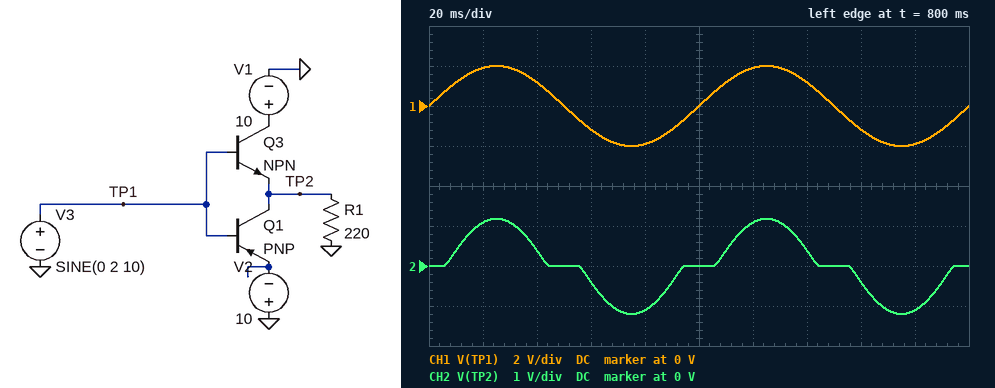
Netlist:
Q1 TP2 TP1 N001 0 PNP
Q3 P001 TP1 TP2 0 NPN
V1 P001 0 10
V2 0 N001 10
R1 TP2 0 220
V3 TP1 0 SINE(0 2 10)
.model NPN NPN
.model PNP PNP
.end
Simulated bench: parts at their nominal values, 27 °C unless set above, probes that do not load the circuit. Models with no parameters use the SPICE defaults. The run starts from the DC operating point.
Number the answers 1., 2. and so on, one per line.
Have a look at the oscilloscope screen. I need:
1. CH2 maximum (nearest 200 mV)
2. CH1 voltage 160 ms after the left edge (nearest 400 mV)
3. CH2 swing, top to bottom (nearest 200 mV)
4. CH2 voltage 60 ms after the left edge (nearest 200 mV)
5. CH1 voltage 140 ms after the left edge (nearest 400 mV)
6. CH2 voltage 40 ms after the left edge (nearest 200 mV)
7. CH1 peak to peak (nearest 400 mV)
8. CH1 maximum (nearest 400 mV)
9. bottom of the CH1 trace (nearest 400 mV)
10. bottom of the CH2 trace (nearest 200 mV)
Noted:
1. 1.2 V
2. -1.2 V
3. 2.4 V
4. -400 mV
5. 1.2 V
6. 400 mV
7. 4.0 V
8. 2.0 V
9. -2.0 V
10. -1.2 V
